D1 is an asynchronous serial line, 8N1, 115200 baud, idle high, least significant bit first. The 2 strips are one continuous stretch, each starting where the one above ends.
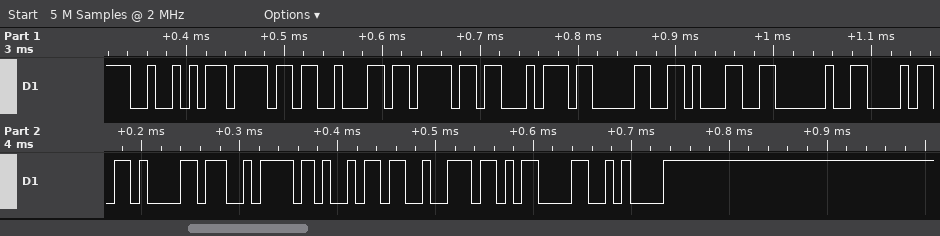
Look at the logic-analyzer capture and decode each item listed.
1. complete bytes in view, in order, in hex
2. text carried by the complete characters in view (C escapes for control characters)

52 6F 62 6F 74 30 31 20 68 61 7A 69 72 0D 0A
"Robot01 hazir\r\n"
